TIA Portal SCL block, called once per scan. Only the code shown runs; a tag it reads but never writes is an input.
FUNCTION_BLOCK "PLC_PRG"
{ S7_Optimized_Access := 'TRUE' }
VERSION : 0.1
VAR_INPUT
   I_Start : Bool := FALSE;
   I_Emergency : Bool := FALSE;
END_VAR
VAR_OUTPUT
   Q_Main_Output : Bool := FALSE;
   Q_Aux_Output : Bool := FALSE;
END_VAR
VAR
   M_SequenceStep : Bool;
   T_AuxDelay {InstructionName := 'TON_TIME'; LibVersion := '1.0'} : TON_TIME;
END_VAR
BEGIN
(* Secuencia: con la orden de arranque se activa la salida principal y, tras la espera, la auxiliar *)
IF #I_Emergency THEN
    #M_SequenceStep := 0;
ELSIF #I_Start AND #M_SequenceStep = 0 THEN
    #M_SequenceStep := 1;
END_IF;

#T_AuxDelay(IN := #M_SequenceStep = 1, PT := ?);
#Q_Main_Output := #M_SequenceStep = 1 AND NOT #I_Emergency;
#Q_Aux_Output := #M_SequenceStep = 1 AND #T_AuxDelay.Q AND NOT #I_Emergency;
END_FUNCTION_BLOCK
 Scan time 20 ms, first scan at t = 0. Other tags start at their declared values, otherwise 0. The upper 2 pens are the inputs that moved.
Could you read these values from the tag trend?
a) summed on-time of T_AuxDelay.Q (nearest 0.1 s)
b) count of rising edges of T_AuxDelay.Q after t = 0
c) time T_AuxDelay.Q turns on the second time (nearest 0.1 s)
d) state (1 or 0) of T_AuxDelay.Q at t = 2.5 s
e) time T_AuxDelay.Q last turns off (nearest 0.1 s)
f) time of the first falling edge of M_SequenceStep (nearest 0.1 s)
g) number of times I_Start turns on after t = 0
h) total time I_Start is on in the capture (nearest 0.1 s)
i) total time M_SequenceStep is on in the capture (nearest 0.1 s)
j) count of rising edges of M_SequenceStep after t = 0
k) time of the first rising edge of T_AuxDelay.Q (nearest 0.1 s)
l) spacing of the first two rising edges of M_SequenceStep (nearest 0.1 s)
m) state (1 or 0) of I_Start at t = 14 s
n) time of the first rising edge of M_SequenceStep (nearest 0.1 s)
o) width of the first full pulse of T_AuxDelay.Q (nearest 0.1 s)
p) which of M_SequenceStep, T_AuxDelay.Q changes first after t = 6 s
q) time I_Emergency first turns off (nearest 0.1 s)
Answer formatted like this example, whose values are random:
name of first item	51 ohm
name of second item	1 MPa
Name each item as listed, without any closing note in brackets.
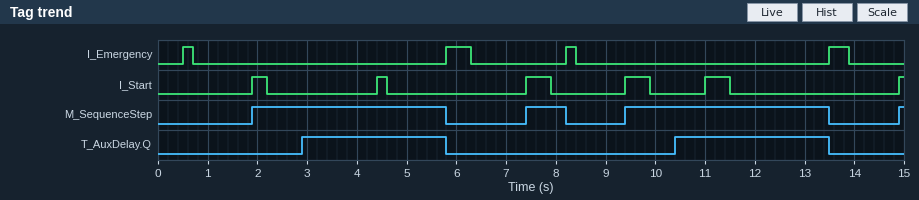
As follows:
summed on-time of T_AuxDelay.Q	6.0 s
count of rising edges of T_AuxDelay.Q after t = 0	2
time T_AuxDelay.Q turns on the second time	10.4 s
state (1 or 0) of T_AuxDelay.Q at t = 2.5 s	0
time T_AuxDelay.Q last turns off	13.5 s
time of the first falling edge of M_SequenceStep	5.8 s
number of times I_Start turns on after t = 0	6
total time I_Start is on in the capture	2.1 s
total time M_SequenceStep is on in the capture	8.9 s
count of rising edges of M_SequenceStep after t = 0	4
time of the first rising edge of T_AuxDelay.Q	2.9 s
spacing of the first two rising edges of M_SequenceStep	5.5 s
state (1 or 0) of I_Start at t = 14 s	0
time of the first rising edge of M_SequenceStep	1.9 s
width of the first full pulse of T_AuxDelay.Q	2.9 s
which of M_SequenceStep, T_AuxDelay.Q changes first after t = 6 s	M_SequenceStep
time I_Emergency first turns off	0.7 s
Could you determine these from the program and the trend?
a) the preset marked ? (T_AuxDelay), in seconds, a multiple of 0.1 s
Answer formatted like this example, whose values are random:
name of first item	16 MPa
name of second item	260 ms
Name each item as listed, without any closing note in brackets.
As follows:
the preset marked ? (T_AuxDelay), in seconds, a multiple of 0.1 s	1.0 s
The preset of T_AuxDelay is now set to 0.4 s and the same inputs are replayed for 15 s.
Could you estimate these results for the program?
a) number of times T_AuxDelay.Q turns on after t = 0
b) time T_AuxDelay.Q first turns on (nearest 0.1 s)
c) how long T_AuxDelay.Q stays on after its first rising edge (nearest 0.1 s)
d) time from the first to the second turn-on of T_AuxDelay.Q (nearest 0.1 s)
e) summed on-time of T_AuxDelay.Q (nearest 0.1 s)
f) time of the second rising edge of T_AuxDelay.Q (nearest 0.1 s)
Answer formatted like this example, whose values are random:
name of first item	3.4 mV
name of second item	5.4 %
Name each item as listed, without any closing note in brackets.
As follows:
number of times T_AuxDelay.Q turns on after t = 0	3
time T_AuxDelay.Q first turns on	2.3 s
how long T_AuxDelay.Q stays on after its first rising edge	3.5 s
time from the first to the second turn-on of T_AuxDelay.Q	5.5 s
summed on-time of T_AuxDelay.Q	7.6 s
time of the second rising edge of T_AuxDelay.Q	7.8 s
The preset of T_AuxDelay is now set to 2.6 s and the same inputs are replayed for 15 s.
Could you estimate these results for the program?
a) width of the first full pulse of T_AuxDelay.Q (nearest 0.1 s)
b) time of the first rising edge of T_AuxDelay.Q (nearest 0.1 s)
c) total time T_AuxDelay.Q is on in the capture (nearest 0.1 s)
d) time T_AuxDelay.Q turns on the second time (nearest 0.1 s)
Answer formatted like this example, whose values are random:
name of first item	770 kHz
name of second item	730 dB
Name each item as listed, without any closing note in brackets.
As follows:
width of the first full pulse of T_AuxDelay.Q	1.3 s
time of the first rising edge of T_AuxDelay.Q	4.5 s
total time T_AuxDelay.Q is on in the capture	2.8 s
time T_AuxDelay.Q turns on the second time	12.0 s
